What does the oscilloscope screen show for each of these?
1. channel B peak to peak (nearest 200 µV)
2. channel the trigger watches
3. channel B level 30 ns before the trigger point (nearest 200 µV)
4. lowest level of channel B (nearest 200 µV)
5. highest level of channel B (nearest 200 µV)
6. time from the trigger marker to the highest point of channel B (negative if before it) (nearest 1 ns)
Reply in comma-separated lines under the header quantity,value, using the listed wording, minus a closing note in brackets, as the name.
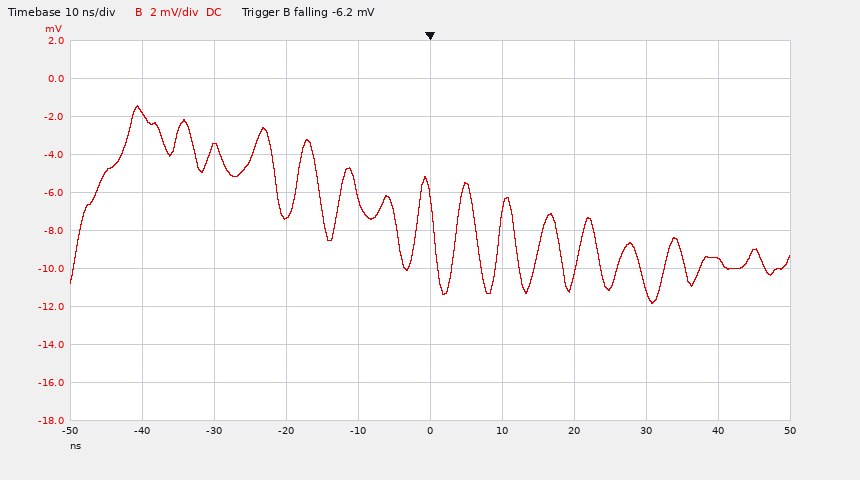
quantity,value
channel B peak to peak,10.4 mV
channel the trigger watches,channel B
channel B level 30 ns before the trigger point,-3.6 mV
lowest level of channel B,-11.8 mV
highest level of channel B,-1.4 mV
time from the trigger marker to the highest point of channel B (negative if before it),-41 ns
